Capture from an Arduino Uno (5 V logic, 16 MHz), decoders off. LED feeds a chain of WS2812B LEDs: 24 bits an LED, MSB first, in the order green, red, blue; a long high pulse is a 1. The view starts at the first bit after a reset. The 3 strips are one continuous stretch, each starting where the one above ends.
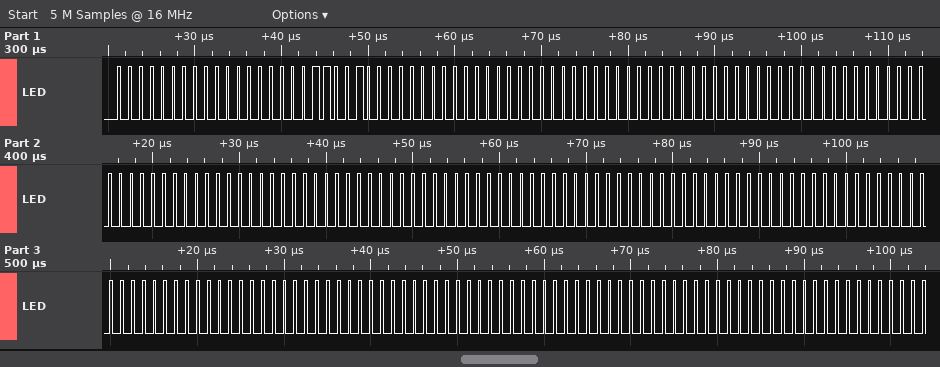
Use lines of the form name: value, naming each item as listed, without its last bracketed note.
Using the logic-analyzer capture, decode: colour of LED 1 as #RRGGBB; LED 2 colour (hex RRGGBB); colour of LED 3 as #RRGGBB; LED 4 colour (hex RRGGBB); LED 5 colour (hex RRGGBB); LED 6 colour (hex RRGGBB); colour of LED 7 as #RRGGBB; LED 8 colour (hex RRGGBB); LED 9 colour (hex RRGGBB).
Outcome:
colour of LED 1 as #RRGGBB: #000032
LED 2 colour: #000000
colour of LED 3 as #RRGGBB: #000000
LED 4 colour: #000000
LED 5 colour: #000000
LED 6 colour: #000000
colour of LED 7 as #RRGGBB: #000000
LED 8 colour: #000000
LED 9 colour: #000000
